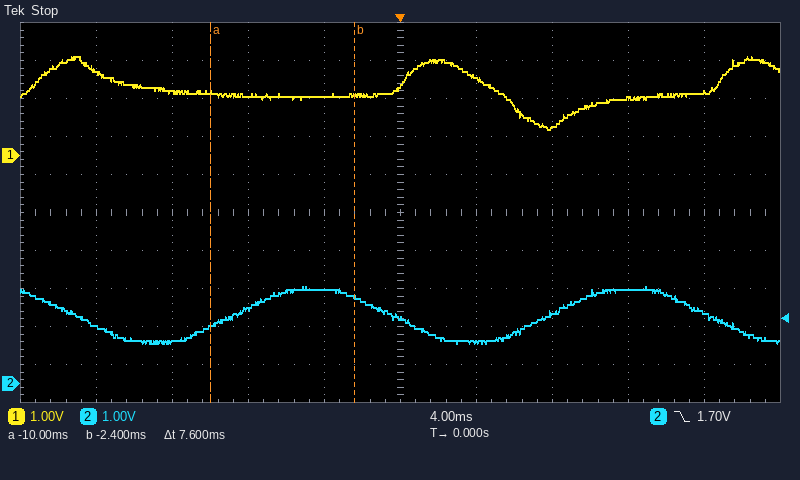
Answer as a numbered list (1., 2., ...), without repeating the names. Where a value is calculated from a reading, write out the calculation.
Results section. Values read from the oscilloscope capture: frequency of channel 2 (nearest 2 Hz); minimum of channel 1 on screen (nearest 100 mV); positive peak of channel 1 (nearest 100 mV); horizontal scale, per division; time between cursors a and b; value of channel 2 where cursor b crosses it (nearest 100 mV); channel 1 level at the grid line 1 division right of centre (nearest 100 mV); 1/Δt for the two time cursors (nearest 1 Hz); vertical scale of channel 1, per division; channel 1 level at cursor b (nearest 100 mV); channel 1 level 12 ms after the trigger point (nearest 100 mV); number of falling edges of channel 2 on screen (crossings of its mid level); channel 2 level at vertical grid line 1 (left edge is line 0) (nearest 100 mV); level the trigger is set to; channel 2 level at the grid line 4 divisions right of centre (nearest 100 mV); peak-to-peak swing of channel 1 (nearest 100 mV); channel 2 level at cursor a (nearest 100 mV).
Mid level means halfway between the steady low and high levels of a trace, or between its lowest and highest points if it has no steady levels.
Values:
1. 60 Hz
2. 700 mV
3. 2.6 V
4. 4 ms
5. 7.6 ms
6. 2.3 V
7. 2.0 V
8. 1 / 7.6 ms ≈ 132 Hz
9. 1 V
10. 1.6 V
11. 1.5 V
12. 3
13. 1.5 V
14. 1.70 V
15. 1.9 V
16. 2.6 V − (700 mV) = 1.9 V
17. 1.5 V
